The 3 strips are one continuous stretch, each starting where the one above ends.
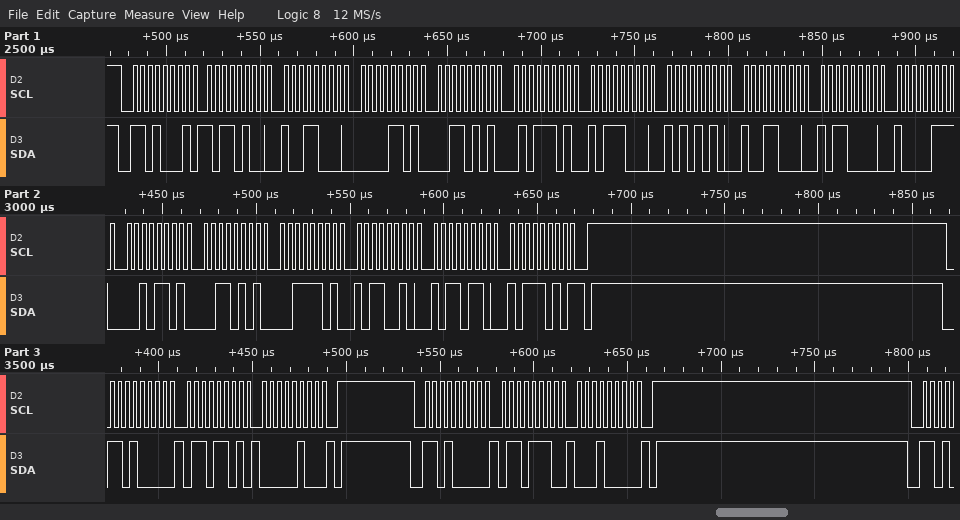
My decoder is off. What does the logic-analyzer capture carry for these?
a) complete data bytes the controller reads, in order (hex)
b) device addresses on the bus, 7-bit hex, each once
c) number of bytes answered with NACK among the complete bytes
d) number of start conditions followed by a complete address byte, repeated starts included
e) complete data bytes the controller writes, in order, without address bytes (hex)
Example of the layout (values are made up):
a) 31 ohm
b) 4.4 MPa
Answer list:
a) B4 98 0D 35 5D B8 AA 98 B0 87 2D 35 3D B2 B6 BA
b) 0x68
c) 1
d) 3
e) 6D 04 6E 10
